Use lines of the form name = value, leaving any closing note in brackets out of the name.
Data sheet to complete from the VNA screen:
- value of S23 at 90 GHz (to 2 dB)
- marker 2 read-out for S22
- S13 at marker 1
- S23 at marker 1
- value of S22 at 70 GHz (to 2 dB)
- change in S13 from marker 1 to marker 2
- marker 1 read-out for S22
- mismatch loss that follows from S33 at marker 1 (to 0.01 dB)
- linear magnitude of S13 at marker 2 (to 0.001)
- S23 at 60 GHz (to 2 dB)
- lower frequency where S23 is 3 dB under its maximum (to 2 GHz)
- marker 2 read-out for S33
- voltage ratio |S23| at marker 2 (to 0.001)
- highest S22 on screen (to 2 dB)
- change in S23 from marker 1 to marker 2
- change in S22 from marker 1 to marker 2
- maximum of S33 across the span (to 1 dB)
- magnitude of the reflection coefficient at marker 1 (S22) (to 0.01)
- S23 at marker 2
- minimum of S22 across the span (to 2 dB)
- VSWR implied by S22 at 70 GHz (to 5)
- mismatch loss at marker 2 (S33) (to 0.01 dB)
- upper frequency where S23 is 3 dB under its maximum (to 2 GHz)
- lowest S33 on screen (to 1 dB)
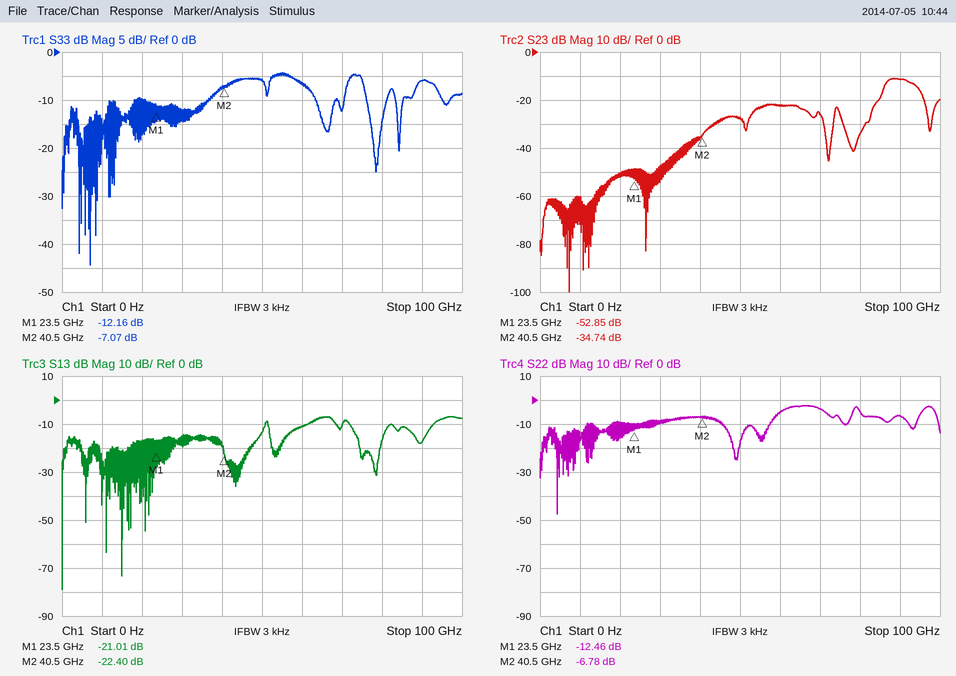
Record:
value of S23 at 90 GHz = -12 dB
marker 2 read-out for S22 = -6.78 dB
S13 at marker 1 = -21.01 dB
S23 at marker 1 = -52.85 dB
value of S22 at 70 GHz = -4 dB
change in S13 from marker 1 to marker 2 = -1.39 dB
marker 1 read-out for S22 = -12.46 dB
mismatch loss that follows from S33 at marker 1 = 0.27 dB
linear magnitude of S13 at marker 2 = 0.076
S23 at 60 GHz = -22 dB
lower frequency where S23 is 3 dB under its maximum = 86 GHz
marker 2 read-out for S33 = -7.07 dB
voltage ratio |S23| at marker 2 = 0.018
highest S22 on screen = -2 dB
change in S23 from marker 1 to marker 2 = 18.11 dB
change in S22 from marker 1 to marker 2 = 5.68 dB
maximum of S33 across the span = -4 dB
magnitude of the reflection coefficient at marker 1 (S22) = 0.24
S23 at marker 2 = -34.74 dB
minimum of S22 across the span = -48 dB
VSWR implied by S22 at 70 GHz = 5
mismatch loss at marker 2 (S33) = 0.95 dB
upper frequency where S23 is 3 dB under its maximum = 94 GHz
lowest S33 on screen = -44 dB
